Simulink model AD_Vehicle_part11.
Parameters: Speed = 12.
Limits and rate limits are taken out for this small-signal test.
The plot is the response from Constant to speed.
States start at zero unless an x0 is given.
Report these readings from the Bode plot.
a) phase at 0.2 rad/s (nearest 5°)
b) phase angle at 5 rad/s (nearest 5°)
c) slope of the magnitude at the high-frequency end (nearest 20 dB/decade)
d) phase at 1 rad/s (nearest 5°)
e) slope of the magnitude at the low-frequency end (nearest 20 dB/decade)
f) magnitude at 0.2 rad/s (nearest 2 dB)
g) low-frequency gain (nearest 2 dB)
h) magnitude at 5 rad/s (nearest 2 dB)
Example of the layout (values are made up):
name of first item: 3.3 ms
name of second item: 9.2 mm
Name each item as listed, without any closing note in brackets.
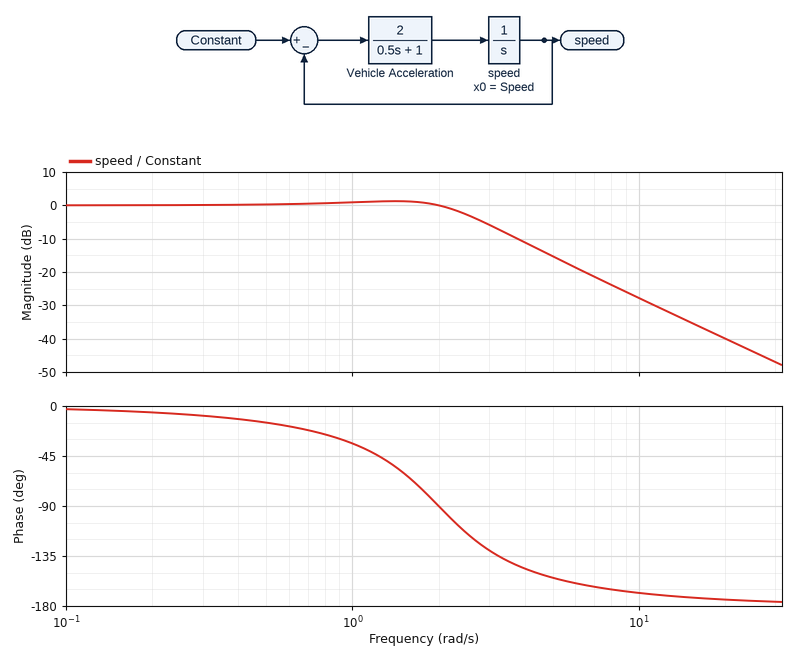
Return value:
phase at 0.2 rad/s: -5°
phase angle at 5 rad/s: -155°
slope of the magnitude at the high-frequency end: -40 dB/decade
phase at 1 rad/s: -35°
slope of the magnitude at the low-frequency end: 0 dB/decade
magnitude at 0.2 rad/s: 0 dB
low-frequency gain: 0 dB
magnitude at 5 rad/s: -16 dB
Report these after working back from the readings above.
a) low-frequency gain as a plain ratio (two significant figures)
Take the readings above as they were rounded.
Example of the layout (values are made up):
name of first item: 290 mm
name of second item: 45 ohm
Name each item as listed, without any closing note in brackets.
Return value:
low-frequency gain as a plain ratio: 1.0
